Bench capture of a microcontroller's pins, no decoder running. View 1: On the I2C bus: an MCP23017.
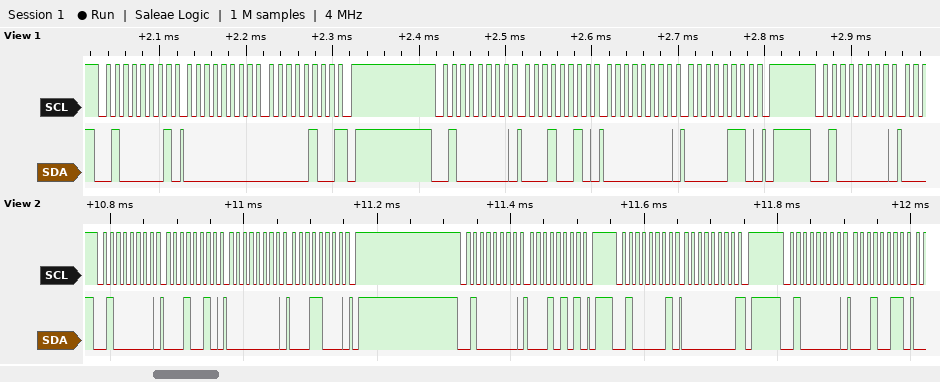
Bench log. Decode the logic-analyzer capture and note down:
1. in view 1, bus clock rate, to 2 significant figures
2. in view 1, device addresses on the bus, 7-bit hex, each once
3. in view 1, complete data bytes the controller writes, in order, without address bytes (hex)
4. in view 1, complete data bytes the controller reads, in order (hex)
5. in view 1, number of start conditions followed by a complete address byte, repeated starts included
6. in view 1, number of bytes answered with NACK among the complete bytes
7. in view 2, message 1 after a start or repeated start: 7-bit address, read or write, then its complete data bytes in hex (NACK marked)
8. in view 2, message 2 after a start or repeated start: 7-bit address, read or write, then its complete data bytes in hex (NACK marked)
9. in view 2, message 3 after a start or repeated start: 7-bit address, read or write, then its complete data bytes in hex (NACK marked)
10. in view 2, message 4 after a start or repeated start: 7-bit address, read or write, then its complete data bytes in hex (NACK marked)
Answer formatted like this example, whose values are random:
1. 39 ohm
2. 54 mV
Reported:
1. 100 kHz
2. 0x20
3. 12 00 06
4. 00 04
5. 3
6. 1
7. 0x20 write: 12 00 18
8. 0x20 write: 15
9. 0x20 read: 00 NACK
10. 0x20 write: 13
